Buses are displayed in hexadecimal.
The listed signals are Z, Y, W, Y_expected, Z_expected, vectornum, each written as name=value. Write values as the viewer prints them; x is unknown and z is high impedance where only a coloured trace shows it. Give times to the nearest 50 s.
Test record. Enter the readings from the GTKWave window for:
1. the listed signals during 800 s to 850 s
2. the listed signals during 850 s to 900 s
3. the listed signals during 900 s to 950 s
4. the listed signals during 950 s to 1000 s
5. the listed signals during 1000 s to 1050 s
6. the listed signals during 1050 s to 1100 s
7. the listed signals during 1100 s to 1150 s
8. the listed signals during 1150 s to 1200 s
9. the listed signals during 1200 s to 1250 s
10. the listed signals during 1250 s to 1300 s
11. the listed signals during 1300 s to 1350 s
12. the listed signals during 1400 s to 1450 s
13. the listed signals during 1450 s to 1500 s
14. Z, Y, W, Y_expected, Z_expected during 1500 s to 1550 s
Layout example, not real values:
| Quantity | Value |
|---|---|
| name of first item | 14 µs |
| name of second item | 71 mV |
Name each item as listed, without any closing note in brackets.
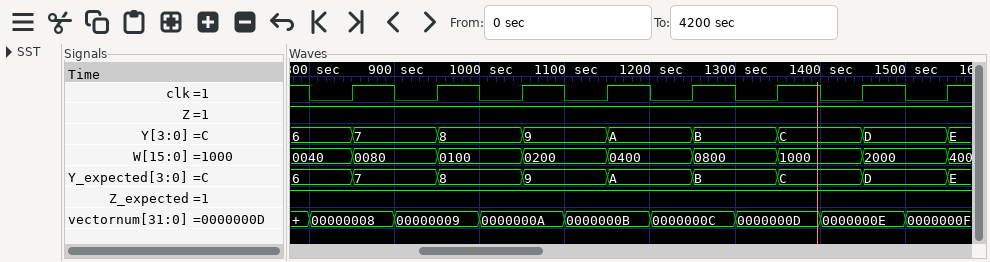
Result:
| Quantity | Value |
|---|---|
| the listed signals during 800 s to 850 s | Z=1, Y=6, W=0040, Y_expected=6, Z_expected=1, vectornum=00000008 |
| the listed signals during 850 s to 900 s | Z=1, Y=7, W=0080, Y_expected=7, Z_expected=1, vectornum=00000008 |
| the listed signals during 900 s to 950 s | Z=1, Y=7, W=0080, Y_expected=7, Z_expected=1, vectornum=00000009 |
| the listed signals during 950 s to 1000 s | Z=1, Y=8, W=0100, Y_expected=8, Z_expected=1, vectornum=00000009 |
| the listed signals during 1000 s to 1050 s | Z=1, Y=8, W=0100, Y_expected=8, Z_expected=1, vectornum=0000000A |
| the listed signals during 1050 s to 1100 s | Z=1, Y=9, W=0200, Y_expected=9, Z_expected=1, vectornum=0000000A |
| the listed signals during 1100 s to 1150 s | Z=1, Y=9, W=0200, Y_expected=9, Z_expected=1, vectornum=0000000B |
| the listed signals during 1150 s to 1200 s | Z=1, Y=A, W=0400, Y_expected=A, Z_expected=1, vectornum=0000000B |
| the listed signals during 1200 s to 1250 s | Z=1, Y=A, W=0400, Y_expected=A, Z_expected=1, vectornum=0000000C |
| the listed signals during 1250 s to 1300 s | Z=1, Y=B, W=0800, Y_expected=B, Z_expected=1, vectornum=0000000C |
| the listed signals during 1300 s to 1350 s | Z=1, Y=B, W=0800, Y_expected=B, Z_expected=1, vectornum=0000000D |
| the listed signals during 1400 s to 1450 s | Z=1, Y=C, W=1000, Y_expected=C, Z_expected=1, vectornum=0000000E |
| the listed signals during 1450 s to 1500 s | Z=1, Y=D, W=2000, Y_expected=D, Z_expected=1, vectornum=0000000E |
| Z, Y, W, Y_expected, Z_expected during 1500 s to 1550 s | Z=1, Y=D, W=2000, Y_expected=D, Z_expected=1 |
